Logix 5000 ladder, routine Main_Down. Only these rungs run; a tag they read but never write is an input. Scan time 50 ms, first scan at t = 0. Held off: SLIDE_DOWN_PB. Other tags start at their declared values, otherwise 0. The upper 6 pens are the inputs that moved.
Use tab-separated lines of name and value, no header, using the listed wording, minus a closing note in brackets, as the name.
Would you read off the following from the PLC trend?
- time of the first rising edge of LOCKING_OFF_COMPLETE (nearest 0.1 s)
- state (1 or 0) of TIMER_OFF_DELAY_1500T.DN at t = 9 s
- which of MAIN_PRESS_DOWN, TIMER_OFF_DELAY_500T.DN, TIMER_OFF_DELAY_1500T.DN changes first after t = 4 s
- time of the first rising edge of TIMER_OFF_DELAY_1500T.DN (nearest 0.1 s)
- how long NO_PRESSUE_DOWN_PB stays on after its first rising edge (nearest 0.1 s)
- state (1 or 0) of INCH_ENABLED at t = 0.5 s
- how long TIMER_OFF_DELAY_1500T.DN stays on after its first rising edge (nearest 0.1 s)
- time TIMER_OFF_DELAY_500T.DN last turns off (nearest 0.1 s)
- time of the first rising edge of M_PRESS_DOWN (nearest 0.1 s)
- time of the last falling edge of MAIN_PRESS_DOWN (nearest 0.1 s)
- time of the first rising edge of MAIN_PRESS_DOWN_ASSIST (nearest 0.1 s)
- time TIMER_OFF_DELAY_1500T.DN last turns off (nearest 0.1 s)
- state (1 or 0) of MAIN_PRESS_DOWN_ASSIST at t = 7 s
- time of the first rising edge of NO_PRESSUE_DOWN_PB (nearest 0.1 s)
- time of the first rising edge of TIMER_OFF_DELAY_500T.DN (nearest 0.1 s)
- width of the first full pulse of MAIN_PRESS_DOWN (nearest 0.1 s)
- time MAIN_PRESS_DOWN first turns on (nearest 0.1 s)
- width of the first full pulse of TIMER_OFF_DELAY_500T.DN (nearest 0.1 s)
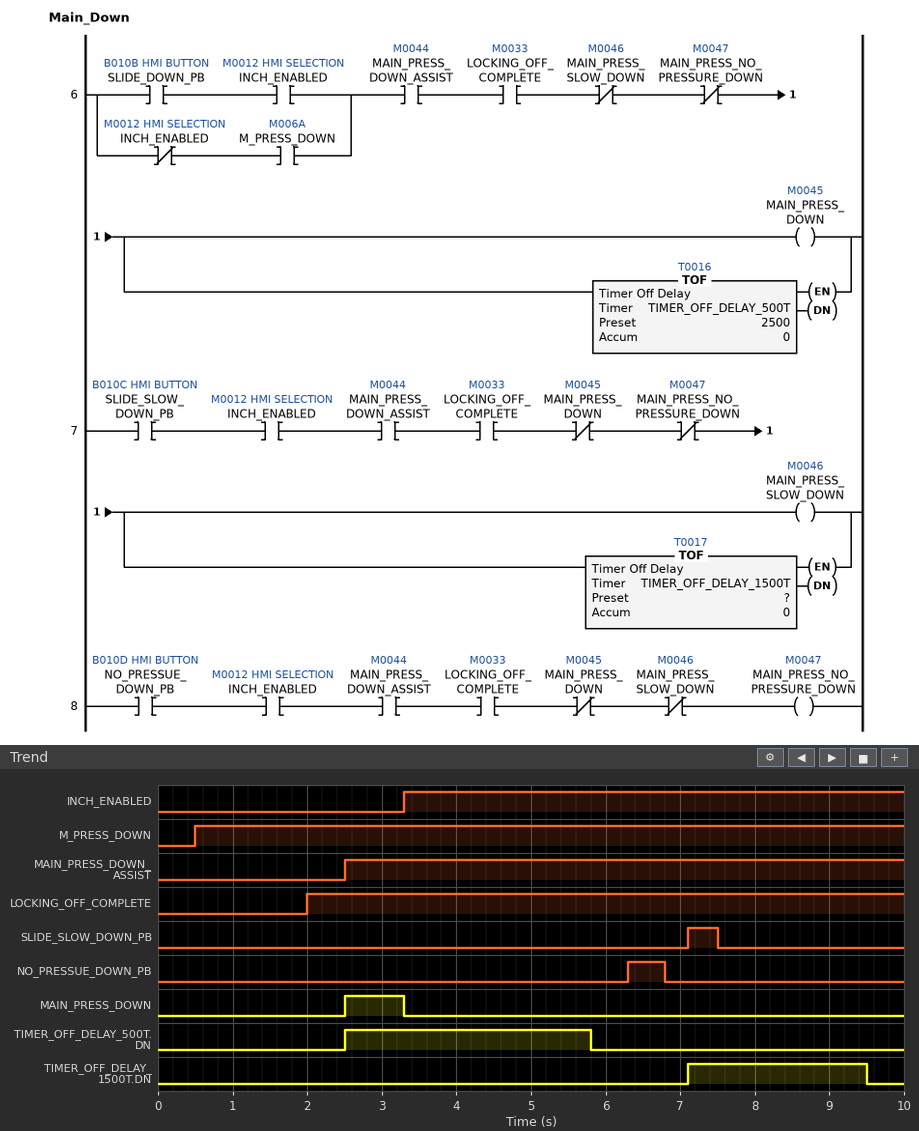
time of the first rising edge of LOCKING_OFF_COMPLETE	2.0 s
state (1 or 0) of TIMER_OFF_DELAY_1500T.DN at t = 9 s	1
which of MAIN_PRESS_DOWN, TIMER_OFF_DELAY_500T.DN, TIMER_OFF_DELAY_1500T.DN changes first after t = 4 s	TIMER_OFF_DELAY_500T.DN
time of the first rising edge of TIMER_OFF_DELAY_1500T.DN	7.1 s
how long NO_PRESSUE_DOWN_PB stays on after its first rising edge	0.5 s
state (1 or 0) of INCH_ENABLED at t = 0.5 s	0
how long TIMER_OFF_DELAY_1500T.DN stays on after its first rising edge	2.4 s
time TIMER_OFF_DELAY_500T.DN last turns off	5.8 s
time of the first rising edge of M_PRESS_DOWN	0.5 s
time of the last falling edge of MAIN_PRESS_DOWN	3.3 s
time of the first rising edge of MAIN_PRESS_DOWN_ASSIST	2.5 s
time TIMER_OFF_DELAY_1500T.DN last turns off	9.5 s
state (1 or 0) of MAIN_PRESS_DOWN_ASSIST at t = 7 s	1
time of the first rising edge of NO_PRESSUE_DOWN_PB	6.3 s
time of the first rising edge of TIMER_OFF_DELAY_500T.DN	2.5 s
width of the first full pulse of MAIN_PRESS_DOWN	0.8 s
time MAIN_PRESS_DOWN first turns on	2.5 s
width of the first full pulse of TIMER_OFF_DELAY_500T.DN	3.3 s
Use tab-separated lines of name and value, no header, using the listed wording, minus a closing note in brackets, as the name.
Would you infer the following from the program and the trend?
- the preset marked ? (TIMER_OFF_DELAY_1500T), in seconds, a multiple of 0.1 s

the preset marked ? (TIMER_OFF_DELAY_1500T), in seconds, a multiple of 0.1 s	2.0 s
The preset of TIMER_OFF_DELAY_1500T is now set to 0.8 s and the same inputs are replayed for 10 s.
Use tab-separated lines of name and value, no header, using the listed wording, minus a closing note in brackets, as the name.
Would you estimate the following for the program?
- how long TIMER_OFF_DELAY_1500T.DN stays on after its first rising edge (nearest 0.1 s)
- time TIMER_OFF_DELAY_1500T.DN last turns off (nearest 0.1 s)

how long TIMER_OFF_DELAY_1500T.DN stays on after its first rising edge	1.2 s
time TIMER_OFF_DELAY_1500T.DN last turns off	8.3 s
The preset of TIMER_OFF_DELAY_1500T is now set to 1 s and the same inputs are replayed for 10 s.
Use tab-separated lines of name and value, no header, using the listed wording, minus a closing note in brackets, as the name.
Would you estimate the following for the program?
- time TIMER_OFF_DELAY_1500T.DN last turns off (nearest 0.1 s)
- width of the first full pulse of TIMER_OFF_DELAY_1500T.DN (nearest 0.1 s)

time TIMER_OFF_DELAY_1500T.DN last turns off	8.5 s
width of the first full pulse of TIMER_OFF_DELAY_1500T.DN	1.4 s
